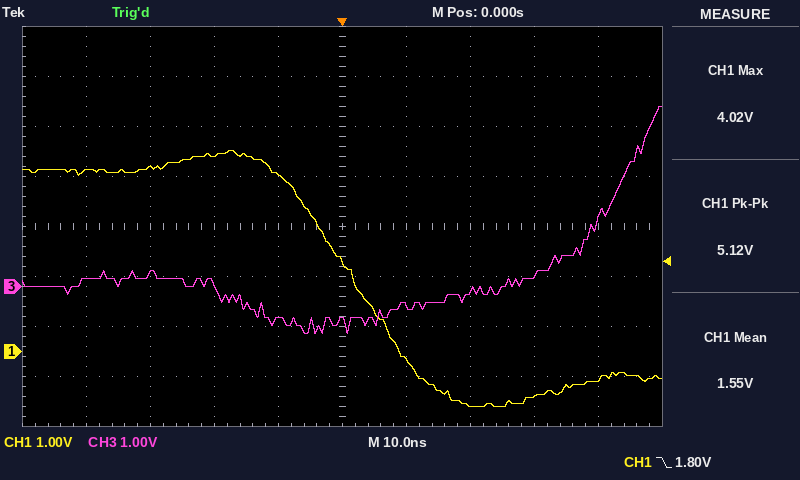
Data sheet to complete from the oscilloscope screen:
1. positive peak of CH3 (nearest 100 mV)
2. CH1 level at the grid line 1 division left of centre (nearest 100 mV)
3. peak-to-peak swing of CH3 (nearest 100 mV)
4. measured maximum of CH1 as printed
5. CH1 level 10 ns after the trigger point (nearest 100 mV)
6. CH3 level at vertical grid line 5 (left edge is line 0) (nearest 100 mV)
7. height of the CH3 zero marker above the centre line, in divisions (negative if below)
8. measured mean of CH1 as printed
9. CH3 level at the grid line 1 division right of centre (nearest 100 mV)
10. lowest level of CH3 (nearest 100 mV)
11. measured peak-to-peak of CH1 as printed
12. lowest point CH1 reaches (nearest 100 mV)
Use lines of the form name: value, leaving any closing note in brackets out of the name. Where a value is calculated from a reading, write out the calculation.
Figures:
positive peak of CH3: 3.6 V
CH1 level at the grid line 1 division left of centre: 3.5 V
peak-to-peak swing of CH3: 3.6 V − (-900 mV) = 4.5 V
measured maximum of CH1 as printed: 4.02 V
CH1 level 10 ns after the trigger point: -200 mV
CH3 level at vertical grid line 5 (left edge is line 0): -700 mV
height of the CH3 zero marker above the centre line, in divisions: -1.2 div
measured mean of CH1 as printed: 1.55 V
CH3 level at the grid line 1 division right of centre: -400 mV
lowest level of CH3: -900 mV
measured peak-to-peak of CH1 as printed: 5.12 V
lowest point CH1 reaches: -1.1 V
